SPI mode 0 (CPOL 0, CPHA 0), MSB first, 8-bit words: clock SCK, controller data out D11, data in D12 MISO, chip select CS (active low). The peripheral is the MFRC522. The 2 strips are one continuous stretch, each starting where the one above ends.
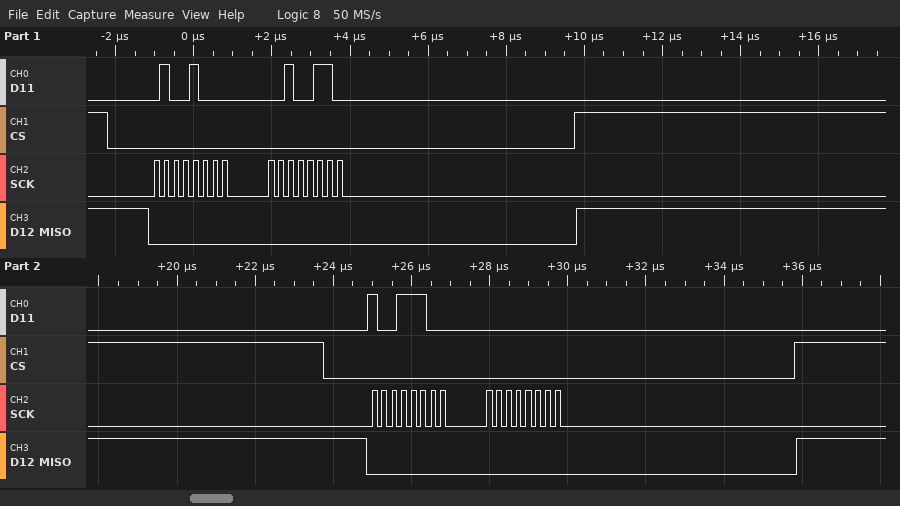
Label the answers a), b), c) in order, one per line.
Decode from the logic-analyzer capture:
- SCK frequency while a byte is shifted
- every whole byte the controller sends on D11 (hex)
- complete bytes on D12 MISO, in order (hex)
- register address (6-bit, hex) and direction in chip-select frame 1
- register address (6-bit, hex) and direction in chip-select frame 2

a) 4 MHz
b) 48 26 9C 00
c) 00 00 00 00
d) 0x24 write
e) 0x0E read
